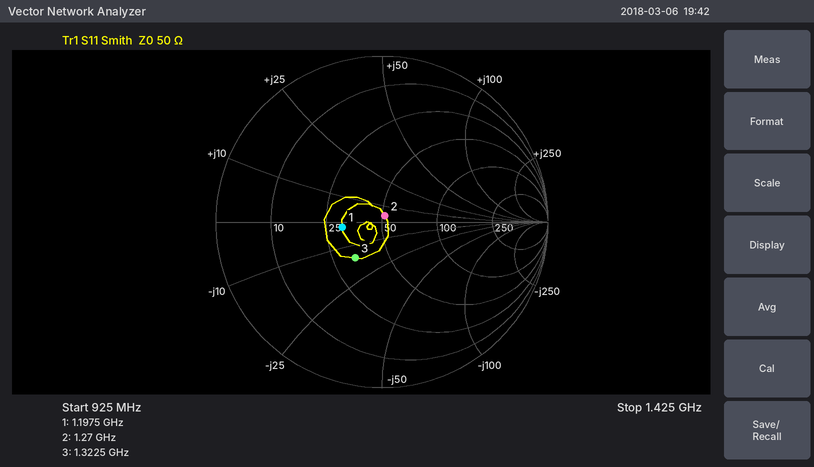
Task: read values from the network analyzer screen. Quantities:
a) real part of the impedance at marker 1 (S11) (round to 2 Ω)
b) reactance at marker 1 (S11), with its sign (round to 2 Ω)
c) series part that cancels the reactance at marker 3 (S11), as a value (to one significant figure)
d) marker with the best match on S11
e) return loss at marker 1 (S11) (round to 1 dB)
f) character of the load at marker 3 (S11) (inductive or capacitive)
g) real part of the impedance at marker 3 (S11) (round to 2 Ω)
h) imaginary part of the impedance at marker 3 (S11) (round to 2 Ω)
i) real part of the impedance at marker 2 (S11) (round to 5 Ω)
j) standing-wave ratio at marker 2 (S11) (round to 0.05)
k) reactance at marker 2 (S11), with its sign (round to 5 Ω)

30 Ω
-2 Ω
2 nH
marker 2
12 dB
capacitive
34 Ω
-16 Ω
50 Ω
1.10
+5 Ω
